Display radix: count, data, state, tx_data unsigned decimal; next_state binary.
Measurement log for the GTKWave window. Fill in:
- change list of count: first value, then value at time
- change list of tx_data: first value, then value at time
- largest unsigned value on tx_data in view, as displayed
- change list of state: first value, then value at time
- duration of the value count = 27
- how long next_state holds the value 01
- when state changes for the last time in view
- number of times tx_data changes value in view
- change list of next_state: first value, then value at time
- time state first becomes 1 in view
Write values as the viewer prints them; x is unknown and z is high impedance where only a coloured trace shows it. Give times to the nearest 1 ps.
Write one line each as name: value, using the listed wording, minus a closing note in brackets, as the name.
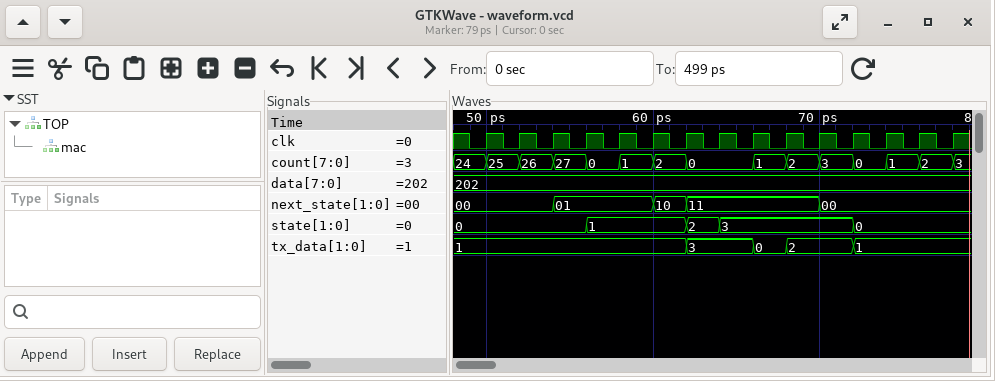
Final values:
change list of count: first value, then value at time: 24, 25 at 50 ps, 26 at 52 ps, 27 at 54 ps, 0 at 56 ps, 1 at 58 ps, 2 at 60 ps, 0 at 62 ps, 1 at 66 ps, 2 at 68 ps, 3 at 70 ps, 0 at 72 ps, 1 at 74 ps, 2 at 76 ps, 3 at 78 ps
change list of tx_data: first value, then value at time: 1, 3 at 62 ps, 0 at 66 ps, 2 at 68 ps, 1 at 72 ps
largest unsigned value on tx_data in view, as displayed: 3
change list of state: first value, then value at time: 0, 1 at 56 ps, 2 at 62 ps, 3 at 64 ps, 0 at 72 ps
duration of the value count = 27: 2 ps
how long next_state holds the value 01: 6 ps
when state changes for the last time in view: 72 ps
number of times tx_data changes value in view: 4
change list of next_state: first value, then value at time: 00, 01 at 54 ps, 10 at 60 ps, 11 at 62 ps, 00 at 70 ps
time state first becomes 1 in view: 56 ps
